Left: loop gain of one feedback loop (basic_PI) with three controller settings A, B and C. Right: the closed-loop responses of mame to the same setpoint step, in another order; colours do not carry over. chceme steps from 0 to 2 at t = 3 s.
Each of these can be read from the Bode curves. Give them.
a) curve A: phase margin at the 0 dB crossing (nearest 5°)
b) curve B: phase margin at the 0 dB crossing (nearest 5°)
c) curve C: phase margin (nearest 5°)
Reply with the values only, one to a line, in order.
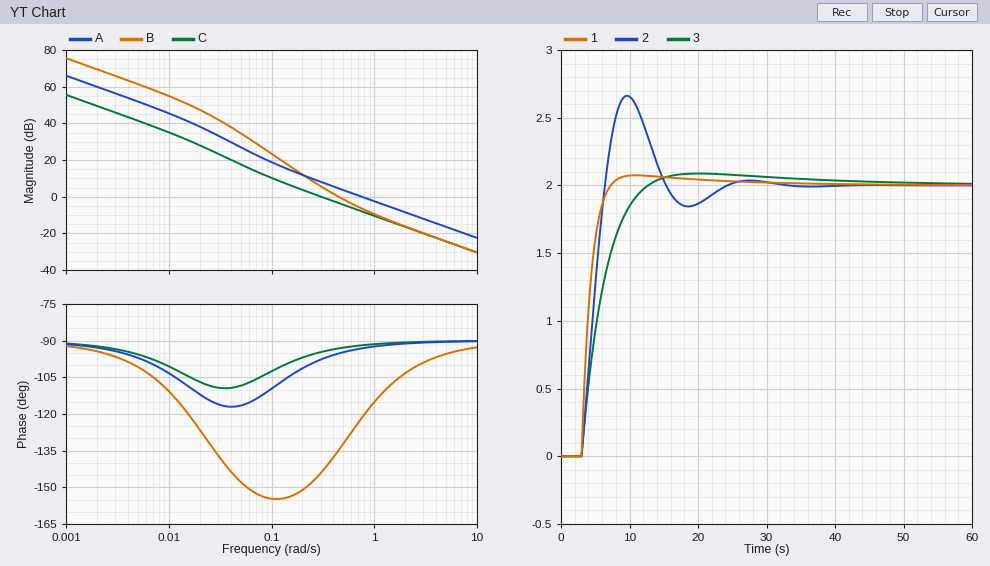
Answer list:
85°
45°
85°
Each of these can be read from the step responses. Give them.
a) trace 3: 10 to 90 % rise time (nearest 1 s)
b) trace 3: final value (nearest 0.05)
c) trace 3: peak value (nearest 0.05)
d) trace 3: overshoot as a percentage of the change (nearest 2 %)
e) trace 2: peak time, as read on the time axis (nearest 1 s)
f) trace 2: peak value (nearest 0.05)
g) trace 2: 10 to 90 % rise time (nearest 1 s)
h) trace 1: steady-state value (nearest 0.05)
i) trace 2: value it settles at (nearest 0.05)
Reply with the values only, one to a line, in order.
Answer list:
6 s
2.00
2.10
4 %
10 s
2.65
3 s
2.00
2.00
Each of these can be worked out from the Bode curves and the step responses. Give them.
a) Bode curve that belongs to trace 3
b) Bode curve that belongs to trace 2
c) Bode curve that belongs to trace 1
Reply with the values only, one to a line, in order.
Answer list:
C
B
A
